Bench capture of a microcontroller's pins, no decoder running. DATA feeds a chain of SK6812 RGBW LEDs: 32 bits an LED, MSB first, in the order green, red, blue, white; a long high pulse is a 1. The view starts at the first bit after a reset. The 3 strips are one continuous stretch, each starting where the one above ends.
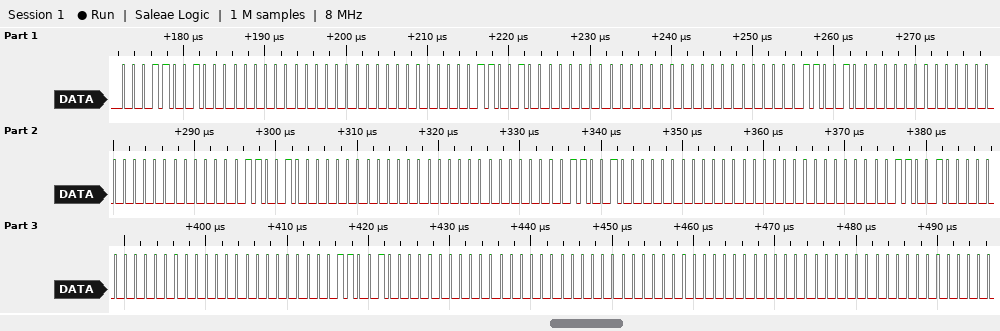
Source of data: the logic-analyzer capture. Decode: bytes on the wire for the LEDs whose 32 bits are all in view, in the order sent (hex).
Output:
19 00 00 00 19 00 00 00 19 00 00 00 19 00 00 00 19 00 00 00 19 00 00 00 19 00 00 00 00 00 00 00
